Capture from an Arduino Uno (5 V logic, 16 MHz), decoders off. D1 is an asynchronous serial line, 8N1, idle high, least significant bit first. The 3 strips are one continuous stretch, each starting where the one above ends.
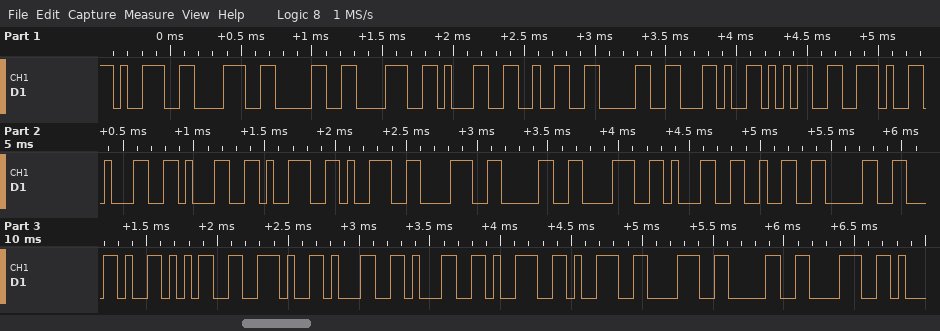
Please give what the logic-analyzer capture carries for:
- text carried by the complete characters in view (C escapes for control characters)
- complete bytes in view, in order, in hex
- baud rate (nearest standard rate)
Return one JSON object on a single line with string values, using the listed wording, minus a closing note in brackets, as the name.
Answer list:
{"text carried by the complete characters in view": "\"9808120,5.1199808120,5.1199808\"", "complete bytes in view, in order, in hex": "39 38 30 38 31 32 30 2C 35 2E 31 31 39 39 38 30 38 31 32 30 2C 35 2E 31 31 39 39 38 30 38", "baud rate": "19200 baud"}
